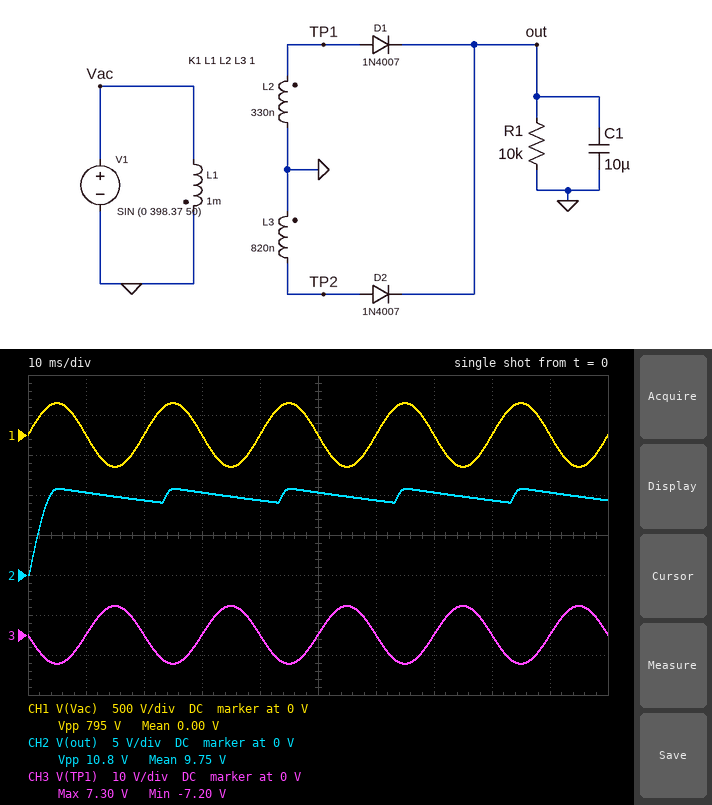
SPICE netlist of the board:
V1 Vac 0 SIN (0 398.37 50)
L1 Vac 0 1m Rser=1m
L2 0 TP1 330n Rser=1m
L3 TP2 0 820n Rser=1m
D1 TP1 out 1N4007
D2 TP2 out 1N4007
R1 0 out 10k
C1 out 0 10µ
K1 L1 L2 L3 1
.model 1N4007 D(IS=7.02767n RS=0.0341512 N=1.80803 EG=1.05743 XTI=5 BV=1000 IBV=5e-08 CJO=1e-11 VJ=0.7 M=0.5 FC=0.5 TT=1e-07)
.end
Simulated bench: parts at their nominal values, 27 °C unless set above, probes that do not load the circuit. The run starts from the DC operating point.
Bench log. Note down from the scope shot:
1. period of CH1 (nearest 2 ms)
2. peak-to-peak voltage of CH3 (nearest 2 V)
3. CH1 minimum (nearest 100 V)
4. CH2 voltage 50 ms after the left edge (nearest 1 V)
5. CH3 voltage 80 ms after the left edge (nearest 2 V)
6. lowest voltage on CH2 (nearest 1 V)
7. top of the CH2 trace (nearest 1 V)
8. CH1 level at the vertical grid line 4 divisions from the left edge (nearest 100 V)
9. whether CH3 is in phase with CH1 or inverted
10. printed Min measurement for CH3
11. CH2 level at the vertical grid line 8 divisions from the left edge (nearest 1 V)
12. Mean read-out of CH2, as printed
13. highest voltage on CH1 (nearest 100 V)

20 ms
14 V
-400 V
10 V
0 V
0 V
11 V
0 V
inverted
-7.20 V
9 V
9.75 V
400 V
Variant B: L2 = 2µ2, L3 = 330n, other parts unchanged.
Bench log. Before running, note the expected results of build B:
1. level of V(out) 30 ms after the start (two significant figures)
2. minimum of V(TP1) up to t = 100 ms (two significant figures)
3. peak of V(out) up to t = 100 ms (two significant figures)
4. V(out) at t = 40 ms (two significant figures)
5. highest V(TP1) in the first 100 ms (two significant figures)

16 V
-19 V
18 V
17 V
19 V
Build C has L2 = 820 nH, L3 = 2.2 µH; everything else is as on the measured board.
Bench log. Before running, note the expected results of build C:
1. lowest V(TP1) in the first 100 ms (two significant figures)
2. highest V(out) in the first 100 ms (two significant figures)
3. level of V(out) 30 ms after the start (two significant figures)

-11 V
18 V
17 V
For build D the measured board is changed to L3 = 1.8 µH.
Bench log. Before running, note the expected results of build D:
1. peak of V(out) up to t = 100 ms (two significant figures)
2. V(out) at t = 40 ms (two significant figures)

16 V
14 V
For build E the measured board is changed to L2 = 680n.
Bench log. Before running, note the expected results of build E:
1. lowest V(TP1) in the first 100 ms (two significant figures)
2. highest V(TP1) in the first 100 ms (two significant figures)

-10 V
10 V
